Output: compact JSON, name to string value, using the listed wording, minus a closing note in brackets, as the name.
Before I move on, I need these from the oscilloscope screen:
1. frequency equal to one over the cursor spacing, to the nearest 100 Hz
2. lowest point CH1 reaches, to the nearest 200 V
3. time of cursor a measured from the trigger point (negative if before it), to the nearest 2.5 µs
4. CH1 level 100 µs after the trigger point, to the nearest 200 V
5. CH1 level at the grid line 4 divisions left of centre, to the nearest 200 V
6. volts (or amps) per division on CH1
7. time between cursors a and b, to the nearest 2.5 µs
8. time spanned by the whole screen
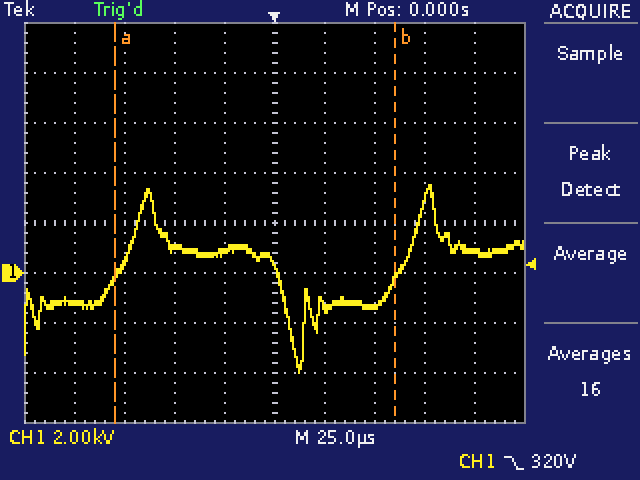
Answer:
{"frequency equal to one over the cursor spacing, to the nearest 100 Hz": "7.1 kHz", "lowest point CH1 reaches, to the nearest 200 V": "-4.0 kV", "time of cursor a measured from the trigger point (negative if before it), to the nearest 2.5 µs": "-80.0 µs", "CH1 level 100 µs after the trigger point, to the nearest 200 V": "800 V", "CH1 level at the grid line 4 divisions left of centre, to the nearest 200 V": "-1.2 kV", "volts (or amps) per division on CH1": "2 kV", "time between cursors a and b, to the nearest 2.5 µs": "140.0 µs", "time spanned by the whole screen": "250 µs"}
